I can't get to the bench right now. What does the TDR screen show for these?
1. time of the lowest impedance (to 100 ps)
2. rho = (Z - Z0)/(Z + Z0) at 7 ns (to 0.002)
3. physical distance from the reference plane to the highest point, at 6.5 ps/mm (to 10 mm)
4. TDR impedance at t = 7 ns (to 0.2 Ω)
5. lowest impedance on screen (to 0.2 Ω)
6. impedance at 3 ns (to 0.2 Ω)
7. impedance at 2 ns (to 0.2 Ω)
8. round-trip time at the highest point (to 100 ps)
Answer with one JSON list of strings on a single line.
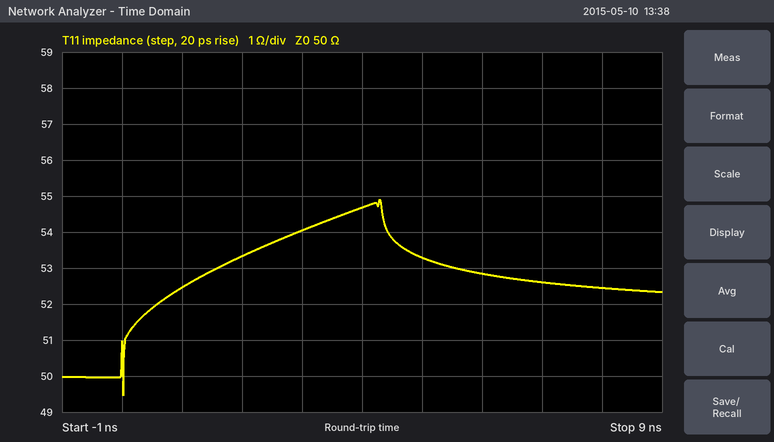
["0.0 ns", "+0.026", "330 mm", "52.6 Ω", "49.4 Ω", "54.0 Ω", "53.4 Ω", "4.3 ns"]
